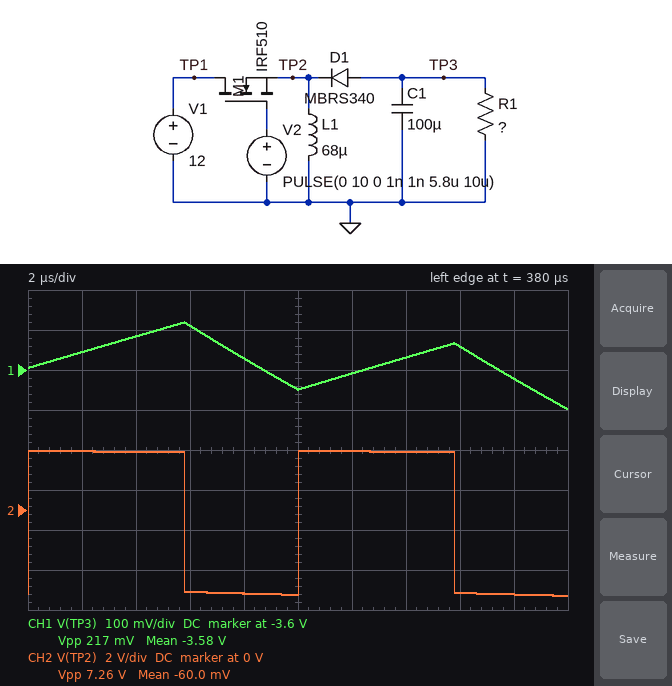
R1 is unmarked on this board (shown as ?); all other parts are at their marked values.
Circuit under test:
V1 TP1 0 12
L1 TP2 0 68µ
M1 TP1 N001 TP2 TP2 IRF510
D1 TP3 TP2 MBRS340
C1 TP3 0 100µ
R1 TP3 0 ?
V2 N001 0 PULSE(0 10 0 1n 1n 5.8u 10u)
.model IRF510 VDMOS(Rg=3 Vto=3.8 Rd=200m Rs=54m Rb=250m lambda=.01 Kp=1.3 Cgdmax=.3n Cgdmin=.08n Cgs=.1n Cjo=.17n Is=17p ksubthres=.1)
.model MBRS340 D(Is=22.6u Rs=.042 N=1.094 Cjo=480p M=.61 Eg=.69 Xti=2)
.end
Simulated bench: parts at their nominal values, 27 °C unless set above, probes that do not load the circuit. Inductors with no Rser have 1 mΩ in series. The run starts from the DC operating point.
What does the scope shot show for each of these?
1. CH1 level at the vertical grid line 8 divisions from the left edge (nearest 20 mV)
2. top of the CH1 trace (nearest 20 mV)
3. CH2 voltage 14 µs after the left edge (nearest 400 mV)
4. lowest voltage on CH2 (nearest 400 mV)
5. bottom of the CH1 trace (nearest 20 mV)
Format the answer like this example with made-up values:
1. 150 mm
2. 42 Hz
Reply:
1. -3.54 V
2. -3.48 V
3. 2.8 V
4. -4.4 V
5. -3.70 V
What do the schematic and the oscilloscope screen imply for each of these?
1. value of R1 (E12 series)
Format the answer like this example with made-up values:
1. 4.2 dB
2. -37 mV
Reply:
1. 1.8 Ω
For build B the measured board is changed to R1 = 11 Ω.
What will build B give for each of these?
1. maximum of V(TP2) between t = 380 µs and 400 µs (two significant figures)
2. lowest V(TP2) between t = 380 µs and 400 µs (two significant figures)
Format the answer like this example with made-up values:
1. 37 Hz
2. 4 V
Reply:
1. 3.4 V
2. -5.7 V
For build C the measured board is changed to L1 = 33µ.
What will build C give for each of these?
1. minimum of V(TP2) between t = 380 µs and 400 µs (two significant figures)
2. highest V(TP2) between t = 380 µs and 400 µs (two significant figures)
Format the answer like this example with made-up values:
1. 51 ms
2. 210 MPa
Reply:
1. -4.7 V
2. 3.1 V
